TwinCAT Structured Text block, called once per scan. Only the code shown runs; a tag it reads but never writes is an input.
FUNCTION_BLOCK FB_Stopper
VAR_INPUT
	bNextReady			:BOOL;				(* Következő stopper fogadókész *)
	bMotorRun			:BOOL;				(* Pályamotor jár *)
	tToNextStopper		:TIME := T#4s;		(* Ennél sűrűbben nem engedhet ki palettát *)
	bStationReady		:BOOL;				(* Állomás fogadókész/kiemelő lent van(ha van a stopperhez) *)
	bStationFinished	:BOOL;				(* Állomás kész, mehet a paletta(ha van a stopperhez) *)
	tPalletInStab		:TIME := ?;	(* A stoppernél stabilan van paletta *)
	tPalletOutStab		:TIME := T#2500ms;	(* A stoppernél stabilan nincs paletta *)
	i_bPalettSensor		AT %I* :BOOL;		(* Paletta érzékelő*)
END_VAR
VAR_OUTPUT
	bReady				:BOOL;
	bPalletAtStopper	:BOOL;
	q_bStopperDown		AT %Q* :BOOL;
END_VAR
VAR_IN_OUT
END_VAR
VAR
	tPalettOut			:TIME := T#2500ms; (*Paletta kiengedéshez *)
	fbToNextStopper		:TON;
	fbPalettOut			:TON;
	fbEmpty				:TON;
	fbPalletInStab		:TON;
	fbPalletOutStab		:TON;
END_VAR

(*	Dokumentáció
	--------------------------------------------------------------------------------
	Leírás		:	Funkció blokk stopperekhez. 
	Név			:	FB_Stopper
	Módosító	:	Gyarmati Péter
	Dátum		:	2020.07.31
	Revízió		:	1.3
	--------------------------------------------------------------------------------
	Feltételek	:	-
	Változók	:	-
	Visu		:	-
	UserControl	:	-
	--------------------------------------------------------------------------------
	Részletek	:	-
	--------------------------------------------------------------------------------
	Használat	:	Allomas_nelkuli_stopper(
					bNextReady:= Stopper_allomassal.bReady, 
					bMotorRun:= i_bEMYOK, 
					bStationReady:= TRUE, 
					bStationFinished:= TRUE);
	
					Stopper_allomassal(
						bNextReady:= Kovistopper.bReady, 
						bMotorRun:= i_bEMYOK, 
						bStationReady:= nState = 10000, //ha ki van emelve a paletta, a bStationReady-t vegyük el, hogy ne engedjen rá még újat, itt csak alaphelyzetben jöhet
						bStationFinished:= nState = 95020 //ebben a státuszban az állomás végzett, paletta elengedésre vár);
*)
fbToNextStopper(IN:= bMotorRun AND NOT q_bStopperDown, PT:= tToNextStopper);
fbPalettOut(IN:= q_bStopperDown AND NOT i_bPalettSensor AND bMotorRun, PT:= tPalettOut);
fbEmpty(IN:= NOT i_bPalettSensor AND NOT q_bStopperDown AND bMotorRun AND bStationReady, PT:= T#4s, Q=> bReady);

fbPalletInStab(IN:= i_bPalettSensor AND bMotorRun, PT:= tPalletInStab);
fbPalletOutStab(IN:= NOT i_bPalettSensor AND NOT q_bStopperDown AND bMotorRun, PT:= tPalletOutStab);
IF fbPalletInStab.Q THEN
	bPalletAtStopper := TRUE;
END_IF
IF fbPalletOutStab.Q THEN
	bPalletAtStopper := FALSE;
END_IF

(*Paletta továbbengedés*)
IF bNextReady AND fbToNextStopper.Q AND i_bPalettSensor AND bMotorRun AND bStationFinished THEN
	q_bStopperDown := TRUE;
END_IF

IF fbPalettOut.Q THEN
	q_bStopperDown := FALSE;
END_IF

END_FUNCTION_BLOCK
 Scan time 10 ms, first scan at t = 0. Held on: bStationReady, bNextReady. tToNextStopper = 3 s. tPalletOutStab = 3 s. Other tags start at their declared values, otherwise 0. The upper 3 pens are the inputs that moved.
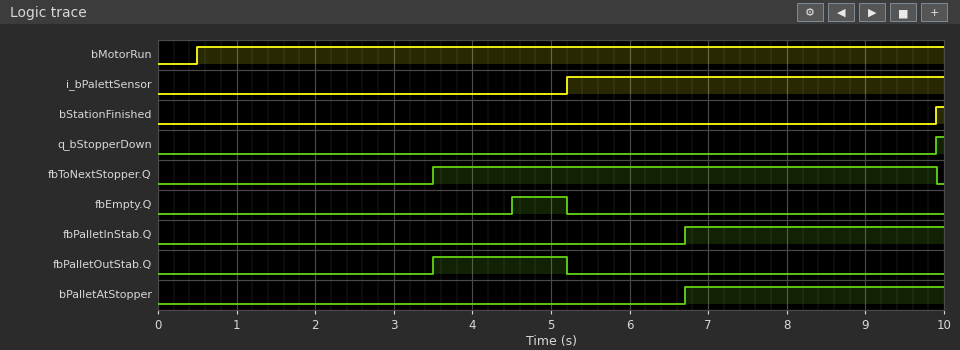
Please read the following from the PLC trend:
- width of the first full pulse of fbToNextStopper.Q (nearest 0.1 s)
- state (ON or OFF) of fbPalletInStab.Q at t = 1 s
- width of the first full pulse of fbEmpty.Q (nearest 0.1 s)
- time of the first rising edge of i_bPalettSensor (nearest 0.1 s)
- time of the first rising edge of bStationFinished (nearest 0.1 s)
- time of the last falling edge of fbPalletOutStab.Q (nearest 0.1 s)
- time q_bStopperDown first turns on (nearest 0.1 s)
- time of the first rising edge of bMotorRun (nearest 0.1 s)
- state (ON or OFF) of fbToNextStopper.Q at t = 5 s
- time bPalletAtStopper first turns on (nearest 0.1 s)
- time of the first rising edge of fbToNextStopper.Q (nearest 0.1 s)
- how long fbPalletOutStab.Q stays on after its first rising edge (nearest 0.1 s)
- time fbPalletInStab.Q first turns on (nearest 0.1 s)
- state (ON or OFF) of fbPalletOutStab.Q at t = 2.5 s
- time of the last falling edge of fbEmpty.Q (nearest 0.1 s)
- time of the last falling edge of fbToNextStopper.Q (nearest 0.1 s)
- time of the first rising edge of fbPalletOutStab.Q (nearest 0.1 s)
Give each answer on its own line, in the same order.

6.4 s
OFF
0.7 s
5.2 s
9.9 s
5.2 s
9.9 s
0.5 s
ON
6.7 s
3.5 s
1.7 s
6.7 s
OFF
5.2 s
9.9 s
3.5 s
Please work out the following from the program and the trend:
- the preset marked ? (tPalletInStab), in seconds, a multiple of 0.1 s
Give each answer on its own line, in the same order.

1.5 s
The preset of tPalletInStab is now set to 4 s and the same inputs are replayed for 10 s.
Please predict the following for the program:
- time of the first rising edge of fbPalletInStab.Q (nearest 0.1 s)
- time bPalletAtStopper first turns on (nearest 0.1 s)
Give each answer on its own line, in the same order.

9.2 s
9.2 s
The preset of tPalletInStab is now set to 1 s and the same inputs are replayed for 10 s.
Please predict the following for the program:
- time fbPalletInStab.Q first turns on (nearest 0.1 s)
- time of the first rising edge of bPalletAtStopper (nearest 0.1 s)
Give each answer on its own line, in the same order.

6.2 s
6.2 s
